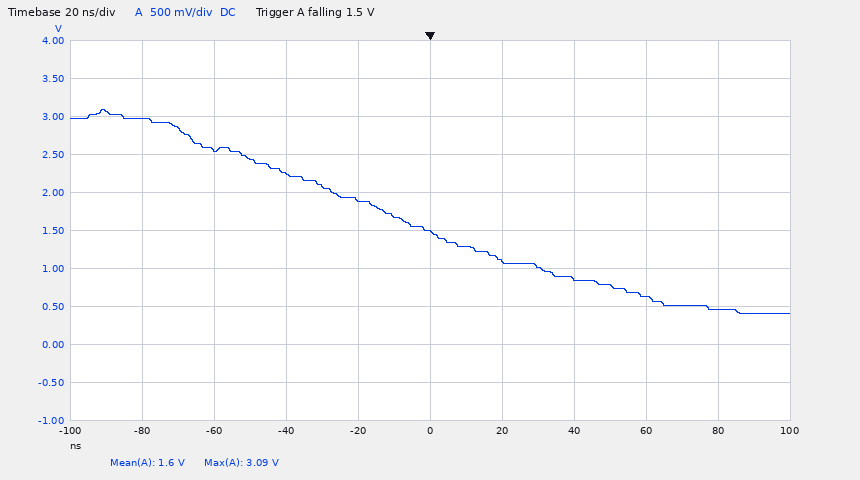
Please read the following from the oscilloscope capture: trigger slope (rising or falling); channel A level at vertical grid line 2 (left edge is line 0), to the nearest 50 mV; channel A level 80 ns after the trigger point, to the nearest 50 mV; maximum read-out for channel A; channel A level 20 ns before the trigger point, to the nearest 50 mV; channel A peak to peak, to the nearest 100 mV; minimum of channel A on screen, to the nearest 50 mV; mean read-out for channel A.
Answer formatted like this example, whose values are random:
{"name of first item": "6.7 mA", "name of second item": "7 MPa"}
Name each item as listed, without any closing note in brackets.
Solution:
{"trigger slope": "falling", "channel A level at vertical grid line 2 (left edge is line 0), to the nearest 50 mV": "2.55 V", "channel A level 80 ns after the trigger point, to the nearest 50 mV": "450 mV", "maximum read-out for channel A": "3.09 V", "channel A level 20 ns before the trigger point, to the nearest 50 mV": "1.90 V", "channel A peak to peak, to the nearest 100 mV": "2.70 V", "minimum of channel A on screen, to the nearest 50 mV": "400 mV", "mean read-out for channel A": "1.6 V"}
